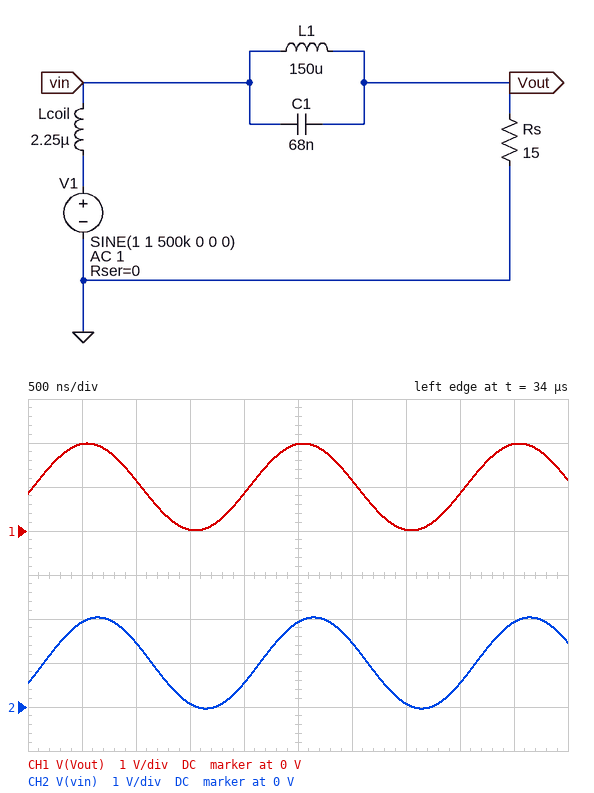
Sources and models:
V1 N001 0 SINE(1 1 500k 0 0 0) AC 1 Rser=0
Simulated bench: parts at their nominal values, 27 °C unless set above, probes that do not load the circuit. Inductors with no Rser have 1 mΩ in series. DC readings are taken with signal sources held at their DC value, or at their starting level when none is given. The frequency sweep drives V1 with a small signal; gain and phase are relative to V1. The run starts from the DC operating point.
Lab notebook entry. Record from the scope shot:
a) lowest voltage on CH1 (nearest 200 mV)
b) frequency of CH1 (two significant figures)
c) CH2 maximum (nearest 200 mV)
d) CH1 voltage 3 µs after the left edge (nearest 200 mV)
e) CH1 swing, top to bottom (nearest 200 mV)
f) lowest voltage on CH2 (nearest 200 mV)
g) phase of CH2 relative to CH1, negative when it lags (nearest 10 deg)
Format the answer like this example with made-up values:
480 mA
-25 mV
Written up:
0 V
500 kHz
2.0 V
1.2 V
2.0 V
0 V
-20 deg
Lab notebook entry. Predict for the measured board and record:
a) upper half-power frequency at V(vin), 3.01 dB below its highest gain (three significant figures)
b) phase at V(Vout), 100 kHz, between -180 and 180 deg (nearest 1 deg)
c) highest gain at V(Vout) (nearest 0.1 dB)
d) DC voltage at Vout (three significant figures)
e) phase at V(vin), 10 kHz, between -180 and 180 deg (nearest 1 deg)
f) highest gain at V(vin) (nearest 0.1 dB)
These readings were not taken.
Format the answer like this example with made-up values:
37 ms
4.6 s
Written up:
1.04 MHz
63 deg
0 dB
1.00 V
0 deg
0.8 dB
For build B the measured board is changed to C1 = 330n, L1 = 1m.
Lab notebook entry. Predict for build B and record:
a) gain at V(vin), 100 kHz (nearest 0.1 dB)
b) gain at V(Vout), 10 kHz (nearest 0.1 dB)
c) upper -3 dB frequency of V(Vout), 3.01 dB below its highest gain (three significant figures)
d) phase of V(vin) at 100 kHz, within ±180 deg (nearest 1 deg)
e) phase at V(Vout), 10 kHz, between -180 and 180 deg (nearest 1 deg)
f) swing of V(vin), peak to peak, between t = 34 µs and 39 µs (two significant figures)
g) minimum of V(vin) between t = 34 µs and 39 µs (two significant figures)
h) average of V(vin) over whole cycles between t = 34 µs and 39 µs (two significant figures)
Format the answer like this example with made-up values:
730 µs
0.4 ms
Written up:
0.2 dB
-22.8 dB
1.09 MHz
-5 deg
86 deg
1.9 V
72 mV
1.0 V
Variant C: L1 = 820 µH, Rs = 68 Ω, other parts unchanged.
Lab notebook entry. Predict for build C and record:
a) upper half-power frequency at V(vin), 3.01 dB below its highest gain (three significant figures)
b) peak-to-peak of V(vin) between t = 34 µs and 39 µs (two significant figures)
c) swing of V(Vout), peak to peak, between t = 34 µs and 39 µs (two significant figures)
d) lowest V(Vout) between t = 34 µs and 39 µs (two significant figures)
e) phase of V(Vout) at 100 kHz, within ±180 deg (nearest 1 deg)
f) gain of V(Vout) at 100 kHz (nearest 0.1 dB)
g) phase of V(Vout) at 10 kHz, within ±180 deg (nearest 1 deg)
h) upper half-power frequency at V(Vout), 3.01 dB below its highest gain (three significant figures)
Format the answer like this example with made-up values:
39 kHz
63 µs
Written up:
4.78 MHz
2.0 V
2.0 V
2.1 mV
19 deg
-0.5 dB
-44 deg
4.84 MHz
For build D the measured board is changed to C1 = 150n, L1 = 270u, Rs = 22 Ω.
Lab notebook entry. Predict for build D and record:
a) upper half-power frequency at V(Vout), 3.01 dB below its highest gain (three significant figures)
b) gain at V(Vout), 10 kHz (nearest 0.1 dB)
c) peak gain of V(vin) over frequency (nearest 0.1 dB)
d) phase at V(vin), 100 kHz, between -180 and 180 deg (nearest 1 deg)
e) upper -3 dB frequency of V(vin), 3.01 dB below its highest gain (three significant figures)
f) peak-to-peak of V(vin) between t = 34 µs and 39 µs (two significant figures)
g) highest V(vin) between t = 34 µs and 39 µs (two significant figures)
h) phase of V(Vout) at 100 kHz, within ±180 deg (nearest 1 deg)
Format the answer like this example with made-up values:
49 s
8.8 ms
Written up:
1.60 MHz
-2.7 dB
0.2 dB
-3 deg
1.53 MHz
2.0 V
2.0 V
24 deg
